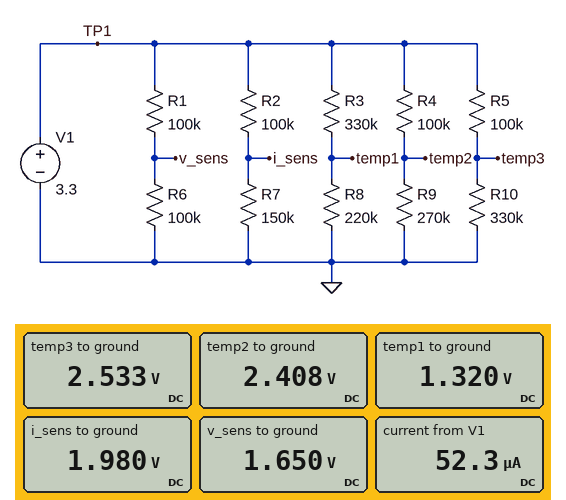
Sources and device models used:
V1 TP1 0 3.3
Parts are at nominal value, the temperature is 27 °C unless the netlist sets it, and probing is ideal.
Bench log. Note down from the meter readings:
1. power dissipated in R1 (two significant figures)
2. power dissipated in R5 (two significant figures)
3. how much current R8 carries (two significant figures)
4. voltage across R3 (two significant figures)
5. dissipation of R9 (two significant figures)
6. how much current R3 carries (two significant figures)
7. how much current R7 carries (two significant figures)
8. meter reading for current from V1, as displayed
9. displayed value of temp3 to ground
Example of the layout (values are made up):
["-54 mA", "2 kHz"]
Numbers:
["27 µW", "5.9 µW", "6.0 µA", "2.0 V", "21 µW", "6.0 µA", "13 µA", "52.3 µA", "2.533 V"]
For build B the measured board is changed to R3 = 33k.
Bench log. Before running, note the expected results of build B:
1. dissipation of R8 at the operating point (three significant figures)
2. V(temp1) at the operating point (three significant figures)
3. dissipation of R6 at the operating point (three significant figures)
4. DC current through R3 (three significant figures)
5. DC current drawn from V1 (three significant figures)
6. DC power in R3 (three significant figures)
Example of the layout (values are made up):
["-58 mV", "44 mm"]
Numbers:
["37.4 µW", "2.87 V", "27.2 µW", "13.0 µA", "59.3 µA", "5.61 µW"]
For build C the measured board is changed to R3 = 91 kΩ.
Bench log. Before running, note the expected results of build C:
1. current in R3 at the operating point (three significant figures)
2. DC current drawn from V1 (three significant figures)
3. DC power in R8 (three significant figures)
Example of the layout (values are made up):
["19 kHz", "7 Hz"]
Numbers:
["10.6 µA", "56.9 µA", "24.8 µW"]
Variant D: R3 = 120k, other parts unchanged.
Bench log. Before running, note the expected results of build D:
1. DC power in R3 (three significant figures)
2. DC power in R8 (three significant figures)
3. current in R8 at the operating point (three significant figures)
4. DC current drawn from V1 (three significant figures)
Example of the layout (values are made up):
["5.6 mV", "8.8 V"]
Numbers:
["11.3 µW", "20.7 µW", "9.71 µA", "56.0 µA"]
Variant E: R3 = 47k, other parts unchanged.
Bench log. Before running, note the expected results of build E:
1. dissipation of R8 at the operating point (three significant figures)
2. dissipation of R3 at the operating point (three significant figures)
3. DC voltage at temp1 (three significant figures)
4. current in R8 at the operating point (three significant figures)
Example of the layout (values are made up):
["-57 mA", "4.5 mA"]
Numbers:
["33.6 µW", "7.18 µW", "2.72 V", "12.4 µA"]
